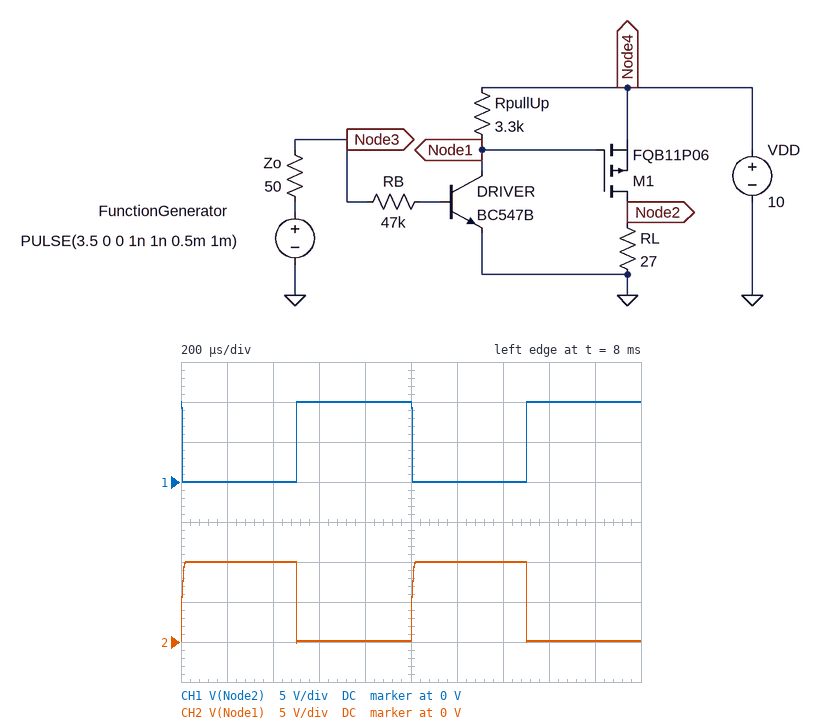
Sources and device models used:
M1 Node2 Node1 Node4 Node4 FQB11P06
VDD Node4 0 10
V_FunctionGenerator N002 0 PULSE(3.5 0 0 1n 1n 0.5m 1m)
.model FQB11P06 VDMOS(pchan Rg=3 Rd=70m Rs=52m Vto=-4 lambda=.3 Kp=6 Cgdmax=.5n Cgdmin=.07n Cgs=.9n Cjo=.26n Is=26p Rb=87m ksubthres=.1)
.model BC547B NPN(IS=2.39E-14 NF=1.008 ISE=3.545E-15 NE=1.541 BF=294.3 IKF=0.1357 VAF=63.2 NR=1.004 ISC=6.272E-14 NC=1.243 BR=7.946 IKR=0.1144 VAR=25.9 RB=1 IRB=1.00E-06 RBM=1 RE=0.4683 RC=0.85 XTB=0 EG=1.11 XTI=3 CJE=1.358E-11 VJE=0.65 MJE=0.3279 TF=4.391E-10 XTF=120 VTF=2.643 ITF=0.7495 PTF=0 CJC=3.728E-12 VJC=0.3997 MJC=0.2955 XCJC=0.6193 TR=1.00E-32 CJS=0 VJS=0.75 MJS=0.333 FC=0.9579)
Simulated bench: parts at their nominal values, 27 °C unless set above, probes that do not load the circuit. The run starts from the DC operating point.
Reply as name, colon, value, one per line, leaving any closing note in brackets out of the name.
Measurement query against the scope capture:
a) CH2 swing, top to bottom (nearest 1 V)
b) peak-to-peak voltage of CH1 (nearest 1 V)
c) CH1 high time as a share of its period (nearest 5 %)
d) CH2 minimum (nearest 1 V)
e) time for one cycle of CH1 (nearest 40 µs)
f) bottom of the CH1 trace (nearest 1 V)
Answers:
CH2 swing, top to bottom: 10 V
peak-to-peak voltage of CH1: 10 V
CH1 high time as a share of its period: 50 %
CH2 minimum: 0 V
time for one cycle of CH1: 1.00 ms
bottom of the CH1 trace: 0 V
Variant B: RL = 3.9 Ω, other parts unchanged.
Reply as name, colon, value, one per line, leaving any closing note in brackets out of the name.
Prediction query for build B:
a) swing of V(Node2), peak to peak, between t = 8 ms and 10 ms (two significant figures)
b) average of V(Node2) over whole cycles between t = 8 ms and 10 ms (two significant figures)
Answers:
swing of V(Node2), peak to peak, between t = 8 ms and 10 ms: 9.6 V
average of V(Node2) over whole cycles between t = 8 ms and 10 ms: 4.9 V
